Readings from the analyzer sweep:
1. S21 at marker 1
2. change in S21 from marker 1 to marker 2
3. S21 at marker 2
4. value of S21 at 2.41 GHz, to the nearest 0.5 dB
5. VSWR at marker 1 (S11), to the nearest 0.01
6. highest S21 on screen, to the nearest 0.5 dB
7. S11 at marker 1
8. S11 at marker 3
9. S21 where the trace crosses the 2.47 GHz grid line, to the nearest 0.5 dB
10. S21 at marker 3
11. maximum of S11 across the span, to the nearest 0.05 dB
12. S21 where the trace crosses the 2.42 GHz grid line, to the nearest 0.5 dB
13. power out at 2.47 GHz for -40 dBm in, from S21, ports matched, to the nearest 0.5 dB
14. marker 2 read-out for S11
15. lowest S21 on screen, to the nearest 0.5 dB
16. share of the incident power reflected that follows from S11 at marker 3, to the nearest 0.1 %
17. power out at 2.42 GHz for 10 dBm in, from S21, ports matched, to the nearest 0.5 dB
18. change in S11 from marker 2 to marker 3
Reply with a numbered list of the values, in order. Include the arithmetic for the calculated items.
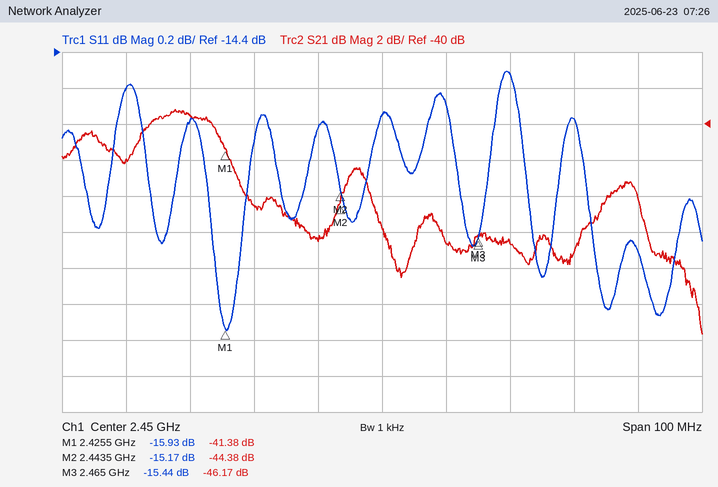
1. -41.38 dB
2. -44.38 − (-41.38) = -3.00 dB
3. -44.38 dB
4. -42.0 dB
5. (1 + 0.1598)/(1 − 0.1598) ≈ 1.38
6. -39.0 dB
7. -15.93 dB
8. -15.44 dB
9. -46.5 dB
10. -46.17 dB
11. -14.50 dB
12. -39.5 dB
13. -40 dBm + (-46.5 dB) = -86.5 dBm
14. -15.17 dB
15. -51.5 dB
16. 10^(-15.44/10) ≈ 2.9 %
17. 10 dBm + (-39.5 dB) = -29.5 dBm
18. -15.44 − (-15.17) = -0.27 dB
